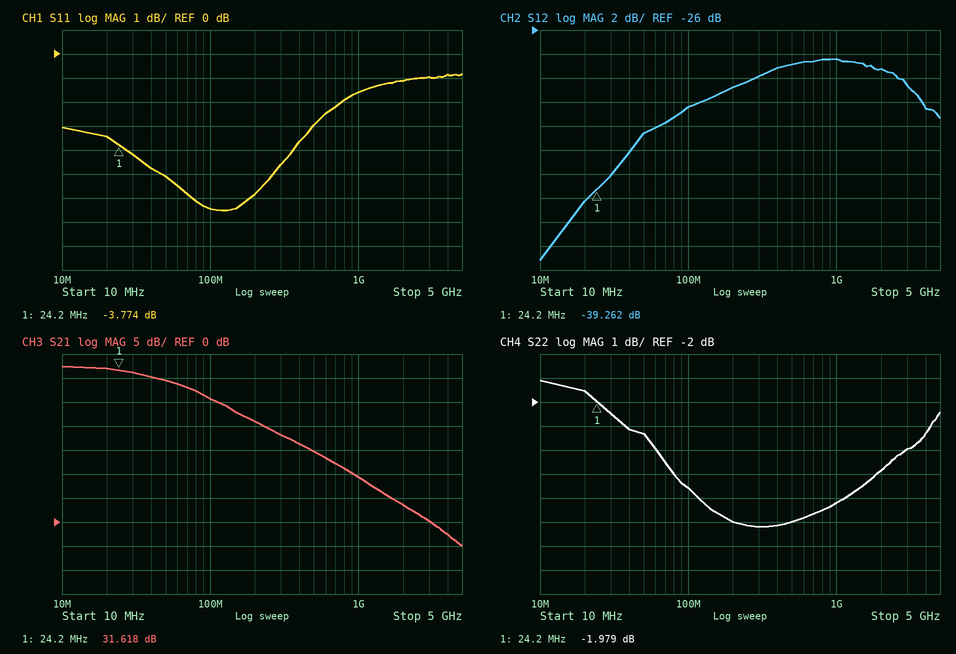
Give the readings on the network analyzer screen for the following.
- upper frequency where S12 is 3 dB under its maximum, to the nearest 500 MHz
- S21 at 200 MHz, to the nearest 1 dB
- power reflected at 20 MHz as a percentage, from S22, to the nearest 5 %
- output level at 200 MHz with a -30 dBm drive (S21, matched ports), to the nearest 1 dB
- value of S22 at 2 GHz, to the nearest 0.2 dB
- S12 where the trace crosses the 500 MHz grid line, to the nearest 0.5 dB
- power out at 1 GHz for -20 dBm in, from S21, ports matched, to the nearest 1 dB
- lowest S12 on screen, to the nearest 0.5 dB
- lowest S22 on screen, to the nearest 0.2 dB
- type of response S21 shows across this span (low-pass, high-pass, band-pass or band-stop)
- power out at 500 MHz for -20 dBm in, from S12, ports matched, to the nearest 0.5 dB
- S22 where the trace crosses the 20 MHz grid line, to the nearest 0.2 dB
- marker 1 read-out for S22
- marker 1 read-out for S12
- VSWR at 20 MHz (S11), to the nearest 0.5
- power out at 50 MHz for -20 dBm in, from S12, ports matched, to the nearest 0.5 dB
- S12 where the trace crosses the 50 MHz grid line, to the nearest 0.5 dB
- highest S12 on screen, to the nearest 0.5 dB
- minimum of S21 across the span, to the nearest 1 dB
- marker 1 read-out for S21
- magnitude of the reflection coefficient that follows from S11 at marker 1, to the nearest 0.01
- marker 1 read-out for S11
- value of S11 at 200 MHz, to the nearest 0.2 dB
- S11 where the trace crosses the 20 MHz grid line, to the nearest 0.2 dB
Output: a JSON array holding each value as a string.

["3.5 GHz", "21 dB", "70 %", "-9 dBm", "-4.8 dB", "-29.0 dB", "-11 dBm", "-45.0 dB", "-7.2 dB", "low-pass", "-49.0 dBm", "-1.6 dB", "-1.979 dB", "-39.262 dB", "5.0", "-54.5 dBm", "-34.5 dB", "-28.5 dB", "-5 dB", "31.618 dB", "0.65", "-3.774 dB", "-5.8 dB", "-3.4 dB"]
